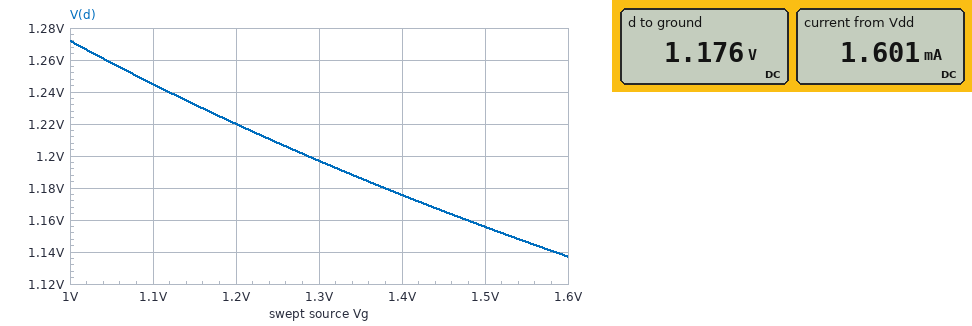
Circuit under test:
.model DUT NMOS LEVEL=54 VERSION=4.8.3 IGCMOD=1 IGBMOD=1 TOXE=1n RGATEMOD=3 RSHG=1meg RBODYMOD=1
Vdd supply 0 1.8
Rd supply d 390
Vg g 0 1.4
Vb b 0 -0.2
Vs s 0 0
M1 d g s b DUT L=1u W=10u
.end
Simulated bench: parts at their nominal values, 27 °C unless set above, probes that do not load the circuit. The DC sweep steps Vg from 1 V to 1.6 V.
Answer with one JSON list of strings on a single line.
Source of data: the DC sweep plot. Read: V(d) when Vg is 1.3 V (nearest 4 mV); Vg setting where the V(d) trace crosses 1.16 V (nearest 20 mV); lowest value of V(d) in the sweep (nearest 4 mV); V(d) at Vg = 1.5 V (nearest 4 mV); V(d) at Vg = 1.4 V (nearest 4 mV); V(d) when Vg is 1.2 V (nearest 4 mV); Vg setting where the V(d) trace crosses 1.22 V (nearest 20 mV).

["1.196 V", "1.48 V", "1.136 V", "1.156 V", "1.176 V", "1.220 V", "1.20 V"]
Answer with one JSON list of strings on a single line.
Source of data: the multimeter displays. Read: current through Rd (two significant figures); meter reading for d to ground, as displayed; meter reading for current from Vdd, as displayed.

["1.6 mA", "1.176 V", "1.601 mA"]
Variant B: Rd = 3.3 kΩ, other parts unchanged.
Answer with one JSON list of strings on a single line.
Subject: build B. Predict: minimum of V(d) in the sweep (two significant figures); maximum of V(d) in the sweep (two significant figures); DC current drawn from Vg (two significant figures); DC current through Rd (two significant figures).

["110 mV", "120 mV", "310 nA", "510 µA"]
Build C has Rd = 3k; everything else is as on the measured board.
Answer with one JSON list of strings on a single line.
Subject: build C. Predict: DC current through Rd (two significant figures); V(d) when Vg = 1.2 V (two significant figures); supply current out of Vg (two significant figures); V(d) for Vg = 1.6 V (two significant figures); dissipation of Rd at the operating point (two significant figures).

["560 µA", "130 mV", "310 nA", "120 mV", "940 µW"]
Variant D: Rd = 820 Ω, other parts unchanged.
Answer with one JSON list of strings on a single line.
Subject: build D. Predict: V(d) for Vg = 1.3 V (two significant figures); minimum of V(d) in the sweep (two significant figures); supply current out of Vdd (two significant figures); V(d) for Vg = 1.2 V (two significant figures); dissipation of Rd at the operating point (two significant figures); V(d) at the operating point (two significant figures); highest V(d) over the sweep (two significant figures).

["600 mV", "510 mV", "1.5 mA", "640 mV", "1.9 mW", "570 mV", "730 mV"]
